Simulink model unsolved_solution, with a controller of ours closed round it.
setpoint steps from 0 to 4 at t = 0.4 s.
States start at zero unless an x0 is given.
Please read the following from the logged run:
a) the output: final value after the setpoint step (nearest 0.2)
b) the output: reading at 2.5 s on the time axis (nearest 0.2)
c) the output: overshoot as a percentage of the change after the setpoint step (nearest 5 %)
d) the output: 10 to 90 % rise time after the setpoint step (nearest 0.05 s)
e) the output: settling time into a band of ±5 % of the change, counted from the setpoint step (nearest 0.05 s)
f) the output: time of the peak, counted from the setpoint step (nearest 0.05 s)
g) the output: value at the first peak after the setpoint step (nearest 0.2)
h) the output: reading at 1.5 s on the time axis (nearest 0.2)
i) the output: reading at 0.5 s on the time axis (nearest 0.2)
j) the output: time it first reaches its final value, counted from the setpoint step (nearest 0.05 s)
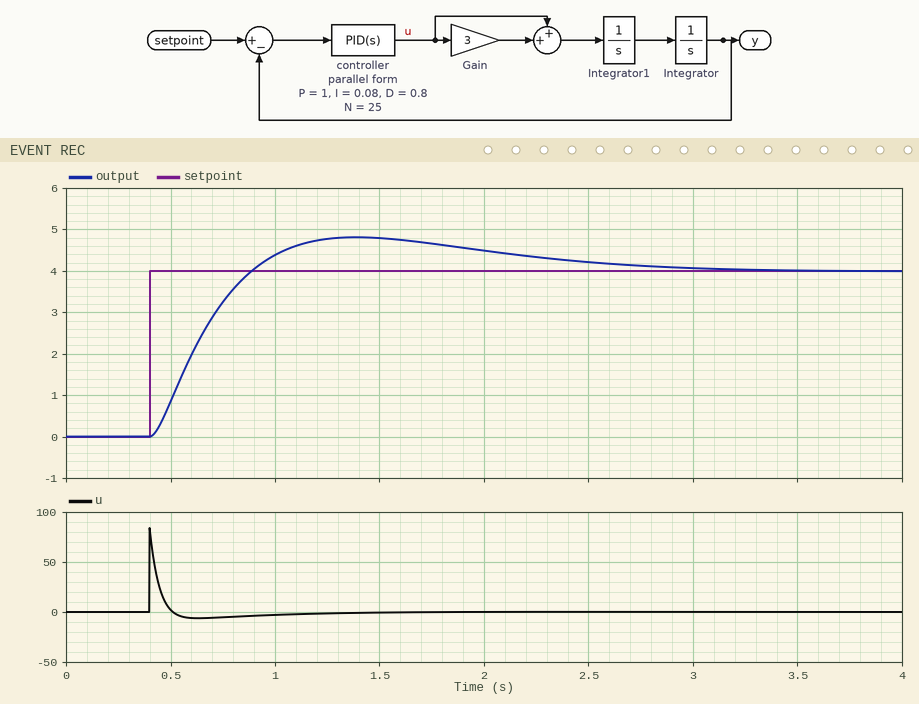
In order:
4.0
4.2
20 %
0.35 s
2.15 s
1.00 s
4.8
4.8
0.8
0.50 s
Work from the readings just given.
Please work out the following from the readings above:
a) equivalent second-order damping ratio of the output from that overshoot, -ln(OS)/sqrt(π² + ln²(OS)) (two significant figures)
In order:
0.46
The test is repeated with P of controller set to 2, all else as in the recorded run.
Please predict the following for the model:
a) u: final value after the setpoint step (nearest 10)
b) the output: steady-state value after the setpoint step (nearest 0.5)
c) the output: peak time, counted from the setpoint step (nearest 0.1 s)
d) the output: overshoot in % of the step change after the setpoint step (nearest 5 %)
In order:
0
4.0
0.8 s
30 %
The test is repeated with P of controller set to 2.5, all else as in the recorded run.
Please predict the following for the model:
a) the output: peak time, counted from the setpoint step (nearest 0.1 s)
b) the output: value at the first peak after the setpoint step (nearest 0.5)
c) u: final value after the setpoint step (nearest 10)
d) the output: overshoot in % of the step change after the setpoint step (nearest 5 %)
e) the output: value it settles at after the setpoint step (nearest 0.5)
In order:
0.7 s
5.5
0
35 %
4.0
